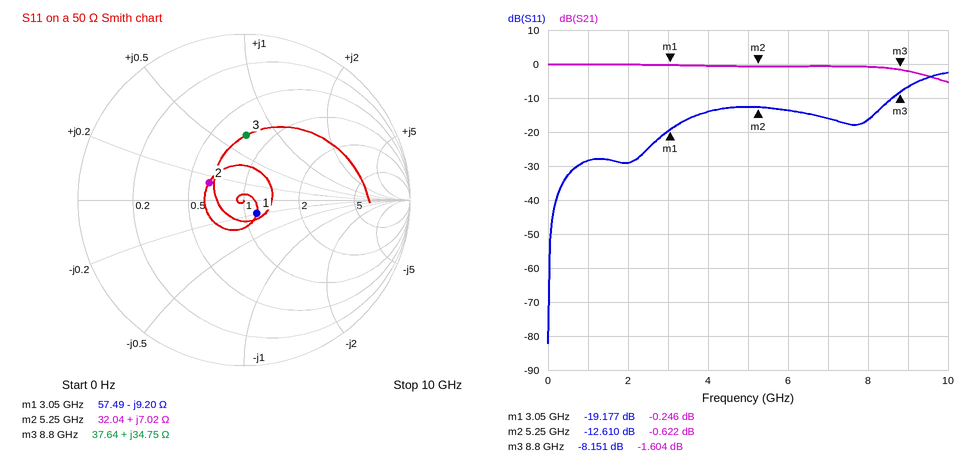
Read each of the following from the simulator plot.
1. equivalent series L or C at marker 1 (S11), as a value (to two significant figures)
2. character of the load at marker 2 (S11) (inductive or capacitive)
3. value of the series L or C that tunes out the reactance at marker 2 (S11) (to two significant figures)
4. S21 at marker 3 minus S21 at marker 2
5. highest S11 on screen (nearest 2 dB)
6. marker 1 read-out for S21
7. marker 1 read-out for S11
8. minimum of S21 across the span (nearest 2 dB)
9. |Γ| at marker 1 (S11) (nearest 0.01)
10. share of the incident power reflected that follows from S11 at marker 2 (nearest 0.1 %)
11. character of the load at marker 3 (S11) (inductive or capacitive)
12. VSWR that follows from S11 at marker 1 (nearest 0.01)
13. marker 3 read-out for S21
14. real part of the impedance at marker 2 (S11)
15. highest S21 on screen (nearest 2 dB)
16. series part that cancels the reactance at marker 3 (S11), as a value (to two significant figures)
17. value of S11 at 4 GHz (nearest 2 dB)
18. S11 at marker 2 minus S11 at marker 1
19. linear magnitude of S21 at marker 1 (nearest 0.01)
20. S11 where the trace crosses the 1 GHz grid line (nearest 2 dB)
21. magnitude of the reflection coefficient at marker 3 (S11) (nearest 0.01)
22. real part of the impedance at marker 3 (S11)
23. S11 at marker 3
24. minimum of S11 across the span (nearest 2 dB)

5.7 pF
inductive
4.3 pF
-0.982 dB
-2 dB
-0.246 dB
-19.177 dB
-6 dB
0.11
5.5 %
inductive
1.25
-1.604 dB
32.04 Ω
0 dB
520 fF
-14 dB
6.567 dB
0.97
-28 dB
0.39
37.64 Ω
-8.151 dB
-82 dB
